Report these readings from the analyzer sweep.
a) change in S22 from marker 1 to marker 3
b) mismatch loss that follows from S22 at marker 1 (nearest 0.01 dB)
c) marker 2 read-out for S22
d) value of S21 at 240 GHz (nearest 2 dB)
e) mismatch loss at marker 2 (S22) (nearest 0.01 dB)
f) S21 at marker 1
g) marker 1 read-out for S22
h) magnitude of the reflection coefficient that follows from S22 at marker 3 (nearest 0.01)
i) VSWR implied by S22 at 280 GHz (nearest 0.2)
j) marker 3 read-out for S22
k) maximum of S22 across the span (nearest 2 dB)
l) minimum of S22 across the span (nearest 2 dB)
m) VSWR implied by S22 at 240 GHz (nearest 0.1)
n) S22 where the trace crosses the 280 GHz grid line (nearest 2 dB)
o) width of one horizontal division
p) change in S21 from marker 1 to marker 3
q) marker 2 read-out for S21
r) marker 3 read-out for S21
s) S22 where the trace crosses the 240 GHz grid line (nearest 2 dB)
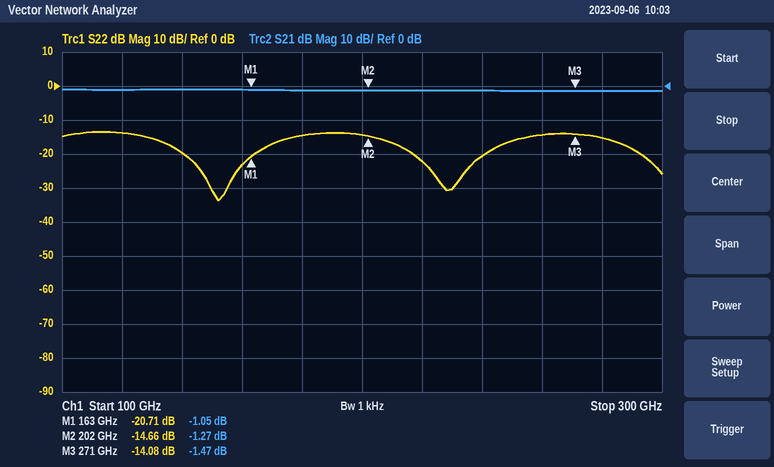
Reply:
6.63 dB
0.04 dB
-14.66 dB
-2 dB
0.15 dB
-1.05 dB
-20.71 dB
0.20
1.4
-14.08 dB
-14 dB
-34 dB
1.2
-16 dB
20 GHz
-0.42 dB
-1.27 dB
-1.47 dB
-20 dB
